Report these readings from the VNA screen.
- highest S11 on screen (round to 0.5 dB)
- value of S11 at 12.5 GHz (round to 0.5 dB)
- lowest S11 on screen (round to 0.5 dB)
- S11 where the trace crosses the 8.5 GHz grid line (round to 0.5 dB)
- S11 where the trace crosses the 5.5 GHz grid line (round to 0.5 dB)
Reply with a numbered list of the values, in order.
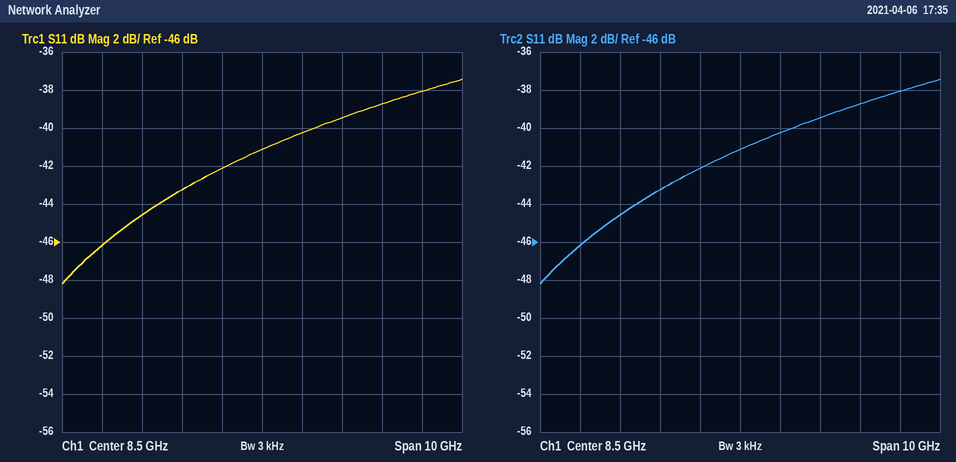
1. -37.5 dB
2. -38.0 dB
3. -48.0 dB
4. -41.0 dB
5. -44.5 dB
